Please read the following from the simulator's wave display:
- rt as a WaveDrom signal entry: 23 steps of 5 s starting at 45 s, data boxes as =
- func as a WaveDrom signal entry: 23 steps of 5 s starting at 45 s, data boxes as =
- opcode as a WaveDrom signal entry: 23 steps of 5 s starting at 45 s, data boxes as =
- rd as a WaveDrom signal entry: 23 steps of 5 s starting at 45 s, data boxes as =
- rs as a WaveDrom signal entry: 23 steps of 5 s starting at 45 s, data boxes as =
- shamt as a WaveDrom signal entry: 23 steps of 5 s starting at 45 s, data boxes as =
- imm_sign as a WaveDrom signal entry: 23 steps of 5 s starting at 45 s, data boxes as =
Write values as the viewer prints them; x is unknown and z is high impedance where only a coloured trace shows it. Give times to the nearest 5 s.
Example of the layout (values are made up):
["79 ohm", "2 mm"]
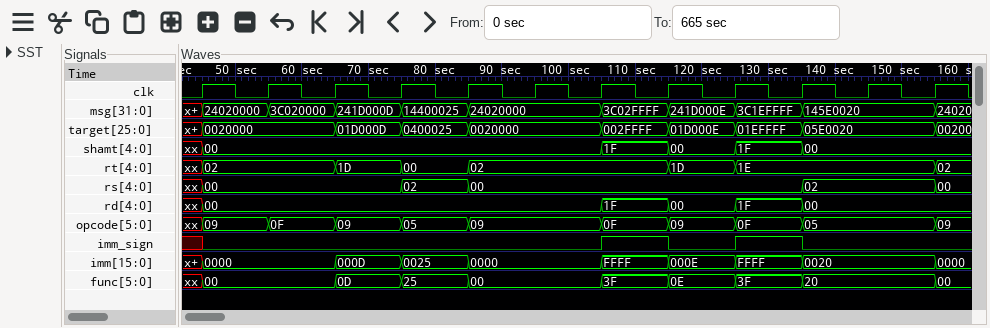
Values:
["{name: 'rt', wave: '=...=.=.=.....=.=.....=', data: '02 1D 00 02 1D 1E 02'}", "{name: 'func', wave: '=...=.=.=...=.=.=.=...=', data: '00 0D 25 00 3F 0E 3F 20 00'}", "{name: 'opcode', wave: '=.=.=.=.=...=.=.=.=...=', data: '09 0F 09 05 09 0F 09 0F 05 09'}", "{name: 'rd', wave: '=...........=.=.=.=....', data: '00 1F 00 1F 00'}", "{name: 'rs', wave: '=.....=.=.........=...=', data: '00 02 00 02 00'}", "{name: 'shamt', wave: '=...........=.=.=.=....', data: '00 1F 00 1F 00'}", "{name: 'imm_sign', wave: '0...........1.0.1.0....'}"]
